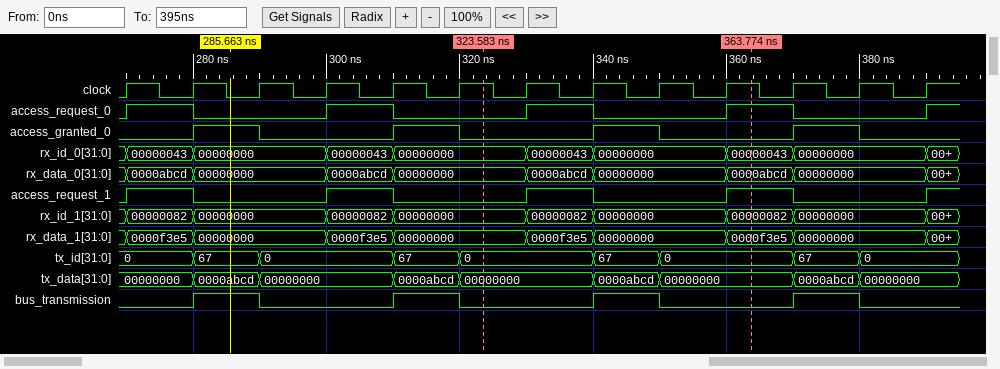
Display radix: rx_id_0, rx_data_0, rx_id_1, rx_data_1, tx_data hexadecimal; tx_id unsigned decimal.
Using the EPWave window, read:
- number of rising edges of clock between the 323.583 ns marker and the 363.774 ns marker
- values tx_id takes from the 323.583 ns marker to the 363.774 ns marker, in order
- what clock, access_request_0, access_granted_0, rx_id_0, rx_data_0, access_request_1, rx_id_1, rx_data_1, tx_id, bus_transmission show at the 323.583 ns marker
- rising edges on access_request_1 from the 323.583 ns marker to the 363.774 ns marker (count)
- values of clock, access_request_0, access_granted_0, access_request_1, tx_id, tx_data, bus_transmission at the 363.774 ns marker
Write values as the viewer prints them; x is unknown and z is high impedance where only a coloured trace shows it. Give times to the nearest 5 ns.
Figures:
4
0, 67, 0
clock=1, access_request_0=0, access_granted_0=0, rx_id_0=00000000, rx_data_0=00000000, access_request_1=0, rx_id_1=00000000, rx_data_1=00000000, tx_id=0, bus_transmission=0
2
clock=1, access_request_0=1, access_granted_0=0, access_request_1=1, tx_id=0, tx_data=00000000, bus_transmission=0
